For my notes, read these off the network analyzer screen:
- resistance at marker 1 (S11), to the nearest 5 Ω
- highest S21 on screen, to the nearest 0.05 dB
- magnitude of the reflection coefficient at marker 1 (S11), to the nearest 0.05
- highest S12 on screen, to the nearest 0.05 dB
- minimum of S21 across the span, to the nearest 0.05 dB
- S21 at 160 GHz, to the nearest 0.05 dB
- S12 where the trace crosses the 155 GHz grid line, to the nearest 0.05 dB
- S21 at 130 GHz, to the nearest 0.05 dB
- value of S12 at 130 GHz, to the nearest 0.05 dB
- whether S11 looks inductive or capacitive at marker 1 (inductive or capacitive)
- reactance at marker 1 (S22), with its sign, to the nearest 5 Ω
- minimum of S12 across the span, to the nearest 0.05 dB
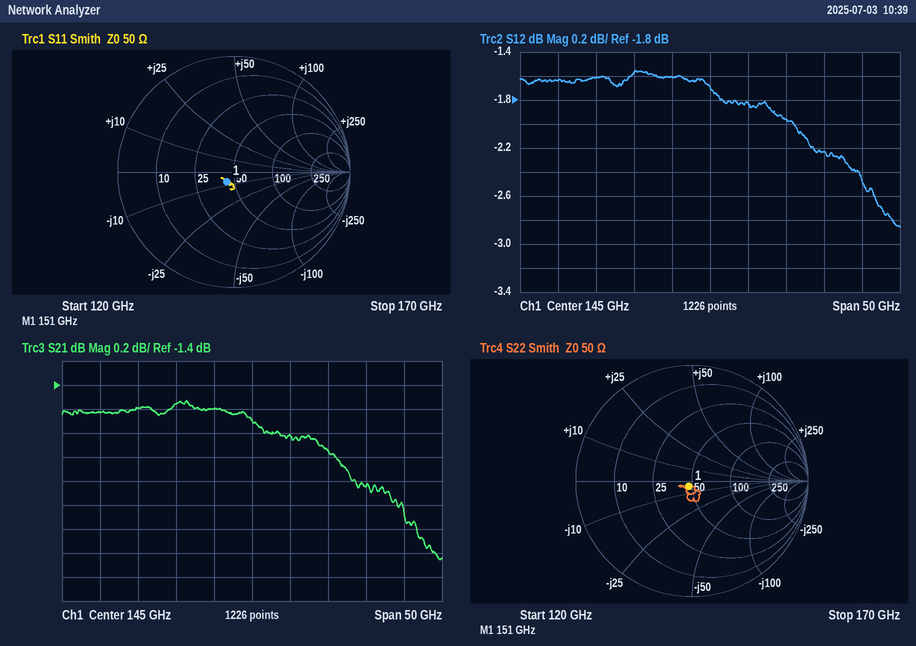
45 Ω
-1.55 dB
0.10
-1.55 dB
-2.85 dB
-2.25 dB
-1.95 dB
-1.60 dB
-1.60 dB
capacitive
-5 Ω
-2.85 dB
